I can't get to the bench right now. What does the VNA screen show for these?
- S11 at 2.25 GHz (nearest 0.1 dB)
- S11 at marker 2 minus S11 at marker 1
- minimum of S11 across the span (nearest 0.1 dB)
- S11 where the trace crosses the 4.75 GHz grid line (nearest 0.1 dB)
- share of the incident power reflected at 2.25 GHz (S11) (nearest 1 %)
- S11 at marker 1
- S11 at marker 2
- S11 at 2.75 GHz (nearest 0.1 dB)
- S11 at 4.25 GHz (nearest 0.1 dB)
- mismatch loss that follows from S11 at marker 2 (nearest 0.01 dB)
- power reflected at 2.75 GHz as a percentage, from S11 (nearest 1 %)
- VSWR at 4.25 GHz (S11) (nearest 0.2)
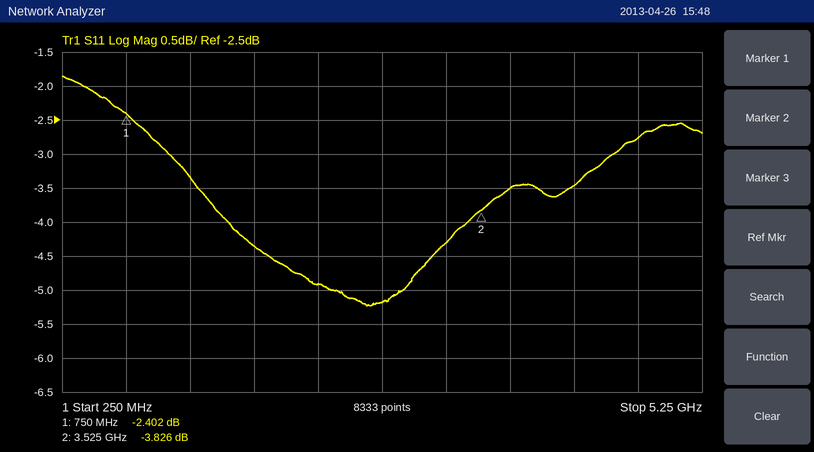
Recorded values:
-4.9 dB
-1.424 dB
-5.2 dB
-2.8 dB
32 %
-2.402 dB
-3.826 dB
-5.2 dB
-3.5 dB
2.32 dB
30 %
5.0
